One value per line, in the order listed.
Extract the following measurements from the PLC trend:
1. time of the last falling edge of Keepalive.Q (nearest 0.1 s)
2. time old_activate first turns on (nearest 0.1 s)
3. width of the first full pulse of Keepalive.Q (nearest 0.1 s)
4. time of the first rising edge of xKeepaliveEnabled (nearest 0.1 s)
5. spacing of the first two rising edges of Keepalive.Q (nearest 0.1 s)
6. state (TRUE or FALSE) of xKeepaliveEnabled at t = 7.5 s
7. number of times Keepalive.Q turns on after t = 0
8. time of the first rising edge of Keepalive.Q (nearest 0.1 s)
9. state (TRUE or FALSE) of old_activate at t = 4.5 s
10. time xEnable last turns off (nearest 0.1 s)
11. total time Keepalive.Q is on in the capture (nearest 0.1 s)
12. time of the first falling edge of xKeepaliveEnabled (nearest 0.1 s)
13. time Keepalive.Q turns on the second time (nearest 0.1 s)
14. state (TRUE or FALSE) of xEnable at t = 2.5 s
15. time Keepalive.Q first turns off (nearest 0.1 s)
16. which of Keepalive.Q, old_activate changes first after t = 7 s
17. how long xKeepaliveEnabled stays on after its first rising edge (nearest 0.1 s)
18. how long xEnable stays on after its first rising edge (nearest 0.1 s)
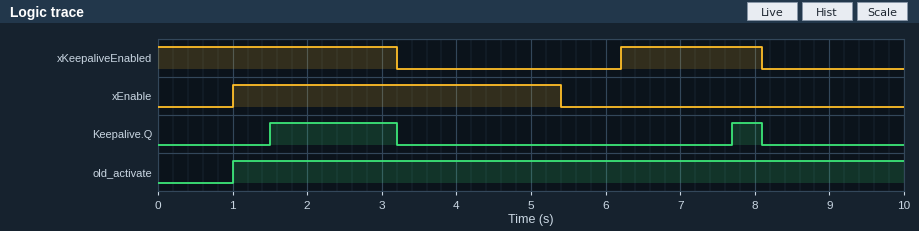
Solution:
8.1 s
1.0 s
1.7 s
6.2 s
6.2 s
TRUE
2
1.5 s
TRUE
5.4 s
2.1 s
3.2 s
7.7 s
TRUE
3.2 s
Keepalive.Q
1.9 s
4.4 s
